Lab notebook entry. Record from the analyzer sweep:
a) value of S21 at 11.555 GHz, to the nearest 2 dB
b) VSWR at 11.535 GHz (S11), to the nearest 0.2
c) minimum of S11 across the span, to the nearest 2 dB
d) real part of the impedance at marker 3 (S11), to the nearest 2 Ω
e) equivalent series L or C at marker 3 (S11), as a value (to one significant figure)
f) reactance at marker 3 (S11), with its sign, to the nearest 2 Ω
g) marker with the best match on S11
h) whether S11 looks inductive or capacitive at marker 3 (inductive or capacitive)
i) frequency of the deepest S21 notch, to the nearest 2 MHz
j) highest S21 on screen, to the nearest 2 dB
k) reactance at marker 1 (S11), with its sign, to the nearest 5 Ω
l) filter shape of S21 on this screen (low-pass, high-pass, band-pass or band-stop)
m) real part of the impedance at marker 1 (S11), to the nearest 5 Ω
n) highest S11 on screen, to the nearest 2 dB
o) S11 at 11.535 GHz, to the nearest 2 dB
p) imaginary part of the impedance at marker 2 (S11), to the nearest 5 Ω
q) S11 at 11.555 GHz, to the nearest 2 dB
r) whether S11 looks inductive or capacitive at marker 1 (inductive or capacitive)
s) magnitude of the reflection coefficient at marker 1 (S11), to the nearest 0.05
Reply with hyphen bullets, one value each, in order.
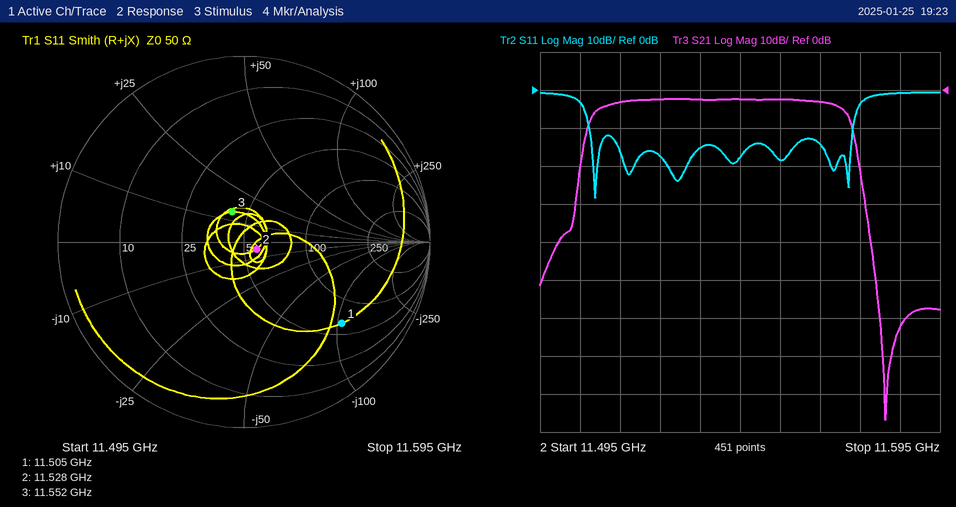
- -2 dB
- 1.4
- -28 dB
- 42 Ω
- 200 pH
- +14 Ω
- marker 2
- inductive
- 11.582 GHz
- -2 dB
- -105 Ω
- band-pass
- 65 Ω
- 0 dB
- -16 dB
- -5 Ω
- -18 dB
- capacitive
- 0.70
